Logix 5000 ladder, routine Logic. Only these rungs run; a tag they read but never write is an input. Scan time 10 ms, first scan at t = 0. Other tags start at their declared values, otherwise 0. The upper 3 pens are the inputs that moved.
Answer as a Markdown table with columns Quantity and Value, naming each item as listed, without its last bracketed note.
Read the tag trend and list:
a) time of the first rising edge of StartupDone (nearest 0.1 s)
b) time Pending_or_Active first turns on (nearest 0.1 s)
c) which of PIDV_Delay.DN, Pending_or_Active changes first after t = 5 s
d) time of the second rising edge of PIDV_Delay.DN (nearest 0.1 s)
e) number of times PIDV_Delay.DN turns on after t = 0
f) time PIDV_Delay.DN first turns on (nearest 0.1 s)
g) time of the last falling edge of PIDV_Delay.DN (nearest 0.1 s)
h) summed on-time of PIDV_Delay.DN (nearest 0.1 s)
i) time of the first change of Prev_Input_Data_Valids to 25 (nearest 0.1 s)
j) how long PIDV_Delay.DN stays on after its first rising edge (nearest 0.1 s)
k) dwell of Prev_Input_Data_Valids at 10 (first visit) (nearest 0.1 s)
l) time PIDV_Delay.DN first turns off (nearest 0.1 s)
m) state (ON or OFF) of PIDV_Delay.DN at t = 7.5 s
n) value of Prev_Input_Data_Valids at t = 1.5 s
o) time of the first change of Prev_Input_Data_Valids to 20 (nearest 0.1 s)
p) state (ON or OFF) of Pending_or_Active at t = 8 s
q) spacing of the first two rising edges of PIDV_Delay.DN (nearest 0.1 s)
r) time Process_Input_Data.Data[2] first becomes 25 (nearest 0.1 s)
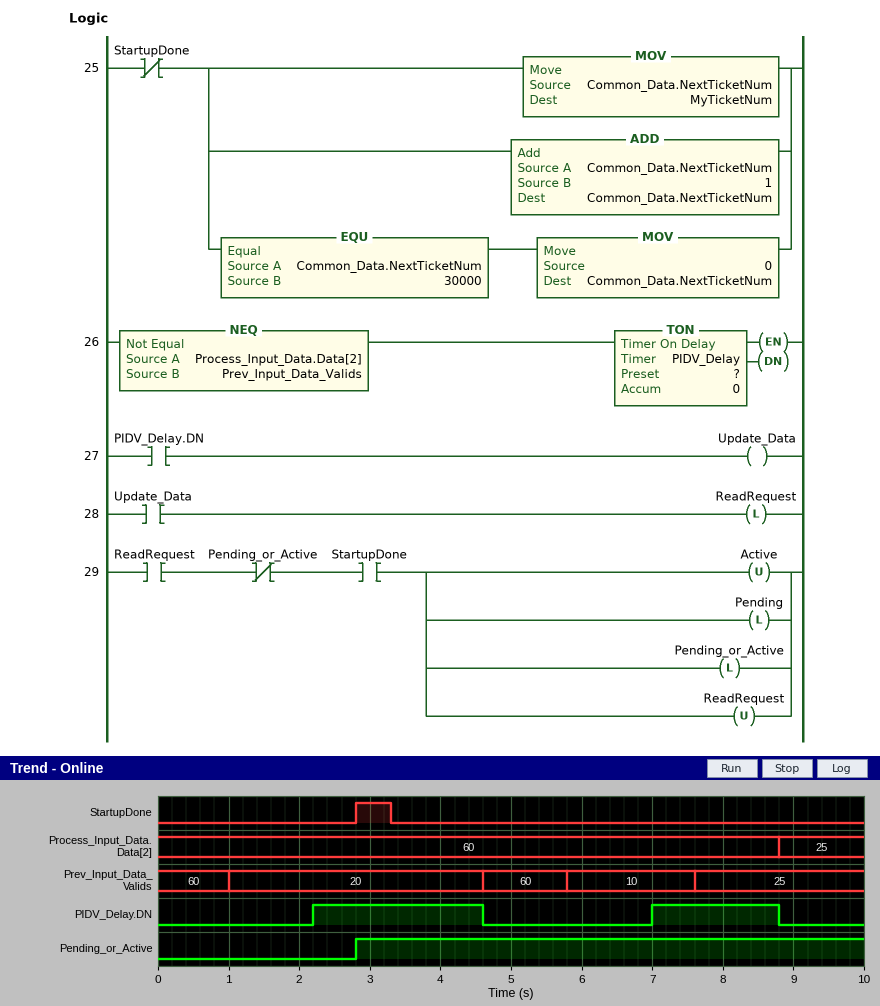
| Quantity | Value |
|---|---|
| time of the first rising edge of StartupDone | 2.8 s |
| time Pending_or_Active first turns on | 2.8 s |
| which of PIDV_Delay.DN, Pending_or_Active changes first after t = 5 s | PIDV_Delay.DN |
| time of the second rising edge of PIDV_Delay.DN | 7.0 s |
| number of times PIDV_Delay.DN turns on after t = 0 | 2 |
| time PIDV_Delay.DN first turns on | 2.2 s |
| time of the last falling edge of PIDV_Delay.DN | 8.8 s |
| summed on-time of PIDV_Delay.DN | 4.2 s |
| time of the first change of Prev_Input_Data_Valids to 25 | 7.6 s |
| how long PIDV_Delay.DN stays on after its first rising edge | 2.4 s |
| dwell of Prev_Input_Data_Valids at 10 (first visit) | 1.8 s |
| time PIDV_Delay.DN first turns off | 4.6 s |
| state (ON or OFF) of PIDV_Delay.DN at t = 7.5 s | ON |
| value of Prev_Input_Data_Valids at t = 1.5 s | 20 |
| time of the first change of Prev_Input_Data_Valids to 20 | 1.0 s |
| state (ON or OFF) of Pending_or_Active at t = 8 s | ON |
| spacing of the first two rising edges of PIDV_Delay.DN | 4.8 s |
| time Process_Input_Data.Data[2] first becomes 25 | 8.8 s |
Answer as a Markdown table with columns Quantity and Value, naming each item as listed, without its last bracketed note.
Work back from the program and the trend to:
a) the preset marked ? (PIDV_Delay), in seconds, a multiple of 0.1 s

| Quantity | Value |
|---|---|
| the preset marked ? (PIDV_Delay), in seconds, a multiple of 0.1 s | 1.2 s |
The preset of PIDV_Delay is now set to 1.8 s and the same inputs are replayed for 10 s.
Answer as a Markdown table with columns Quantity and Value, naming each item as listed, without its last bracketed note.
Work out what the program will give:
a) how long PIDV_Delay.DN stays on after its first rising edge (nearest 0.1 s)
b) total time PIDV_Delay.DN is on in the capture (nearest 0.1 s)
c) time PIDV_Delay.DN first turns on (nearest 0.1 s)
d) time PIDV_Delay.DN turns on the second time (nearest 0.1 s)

| Quantity | Value |
|---|---|
| how long PIDV_Delay.DN stays on after its first rising edge | 1.8 s |
| total time PIDV_Delay.DN is on in the capture | 3.0 s |
| time PIDV_Delay.DN first turns on | 2.8 s |
| time PIDV_Delay.DN turns on the second time | 7.6 s |
